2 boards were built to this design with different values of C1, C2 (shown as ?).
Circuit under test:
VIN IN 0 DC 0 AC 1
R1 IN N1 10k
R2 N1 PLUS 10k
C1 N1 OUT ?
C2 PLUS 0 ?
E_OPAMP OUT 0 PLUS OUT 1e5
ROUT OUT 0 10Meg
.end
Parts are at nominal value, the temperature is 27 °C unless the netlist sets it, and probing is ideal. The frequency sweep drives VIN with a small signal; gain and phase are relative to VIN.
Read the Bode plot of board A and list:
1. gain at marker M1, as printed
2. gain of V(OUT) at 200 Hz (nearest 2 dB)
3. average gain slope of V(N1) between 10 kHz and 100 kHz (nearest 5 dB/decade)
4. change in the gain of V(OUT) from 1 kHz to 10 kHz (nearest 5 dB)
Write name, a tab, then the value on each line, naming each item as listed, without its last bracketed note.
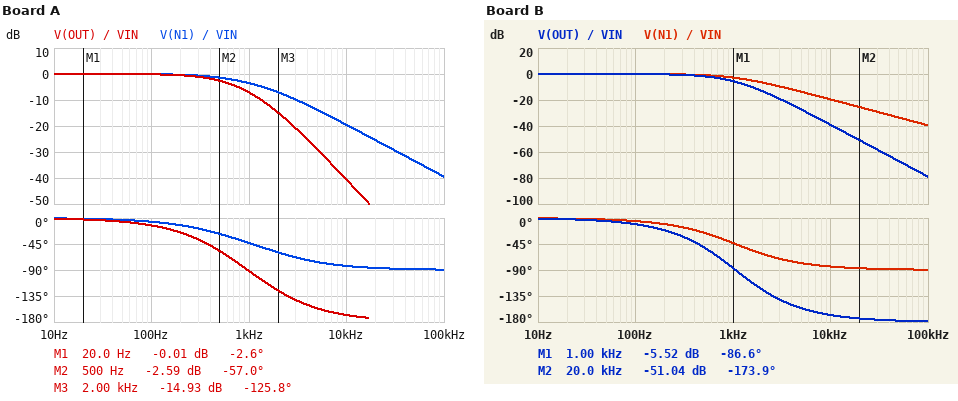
gain at marker M1, as printed	-0.01 dB
gain of V(OUT) at 200 Hz	0 dB
average gain slope of V(N1) between 10 kHz and 100 kHz	-20 dB/decade
change in the gain of V(OUT) from 1 kHz to 10 kHz	-35 dB
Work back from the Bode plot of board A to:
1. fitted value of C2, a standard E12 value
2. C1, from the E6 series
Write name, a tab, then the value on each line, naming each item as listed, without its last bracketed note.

fitted value of C2, a standard E12 value	18 nF
C1, from the E6 series	15 nF
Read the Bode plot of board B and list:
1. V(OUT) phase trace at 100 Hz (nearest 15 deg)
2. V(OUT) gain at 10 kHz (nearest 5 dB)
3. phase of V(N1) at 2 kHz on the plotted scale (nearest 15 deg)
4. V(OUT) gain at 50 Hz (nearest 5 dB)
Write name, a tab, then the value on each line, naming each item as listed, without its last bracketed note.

V(OUT) phase trace at 100 Hz	-15 deg
V(OUT) gain at 10 kHz	-40 dB
phase of V(N1) at 2 kHz on the plotted scale	-60 deg
V(OUT) gain at 50 Hz	0 dB
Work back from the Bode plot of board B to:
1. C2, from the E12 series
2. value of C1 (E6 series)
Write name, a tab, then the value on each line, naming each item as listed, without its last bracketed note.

C2, from the E12 series	15 nF
value of C1	15 nF
